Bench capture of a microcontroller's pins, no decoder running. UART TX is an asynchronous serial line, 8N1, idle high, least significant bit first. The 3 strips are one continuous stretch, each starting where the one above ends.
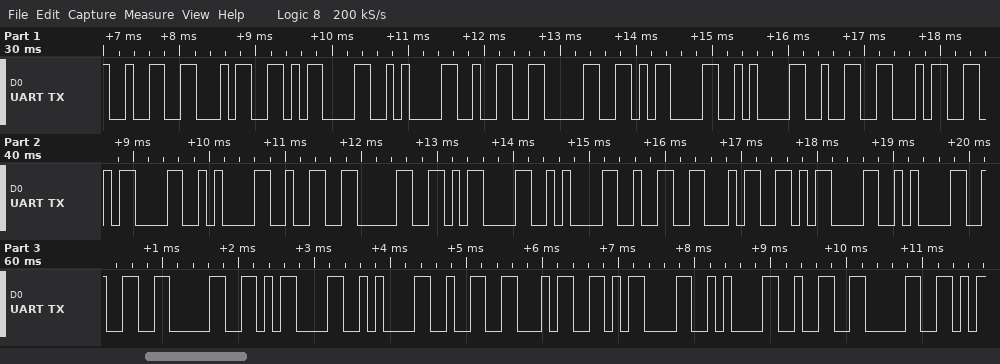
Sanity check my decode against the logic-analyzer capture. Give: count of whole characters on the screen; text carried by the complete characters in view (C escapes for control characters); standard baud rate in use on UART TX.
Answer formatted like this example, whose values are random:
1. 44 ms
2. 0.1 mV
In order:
1. 30
2. "24\r\n20\r\n24\r\n20\r\n24\r\n20\r\n24\r\n20"
3. 9600 baud
